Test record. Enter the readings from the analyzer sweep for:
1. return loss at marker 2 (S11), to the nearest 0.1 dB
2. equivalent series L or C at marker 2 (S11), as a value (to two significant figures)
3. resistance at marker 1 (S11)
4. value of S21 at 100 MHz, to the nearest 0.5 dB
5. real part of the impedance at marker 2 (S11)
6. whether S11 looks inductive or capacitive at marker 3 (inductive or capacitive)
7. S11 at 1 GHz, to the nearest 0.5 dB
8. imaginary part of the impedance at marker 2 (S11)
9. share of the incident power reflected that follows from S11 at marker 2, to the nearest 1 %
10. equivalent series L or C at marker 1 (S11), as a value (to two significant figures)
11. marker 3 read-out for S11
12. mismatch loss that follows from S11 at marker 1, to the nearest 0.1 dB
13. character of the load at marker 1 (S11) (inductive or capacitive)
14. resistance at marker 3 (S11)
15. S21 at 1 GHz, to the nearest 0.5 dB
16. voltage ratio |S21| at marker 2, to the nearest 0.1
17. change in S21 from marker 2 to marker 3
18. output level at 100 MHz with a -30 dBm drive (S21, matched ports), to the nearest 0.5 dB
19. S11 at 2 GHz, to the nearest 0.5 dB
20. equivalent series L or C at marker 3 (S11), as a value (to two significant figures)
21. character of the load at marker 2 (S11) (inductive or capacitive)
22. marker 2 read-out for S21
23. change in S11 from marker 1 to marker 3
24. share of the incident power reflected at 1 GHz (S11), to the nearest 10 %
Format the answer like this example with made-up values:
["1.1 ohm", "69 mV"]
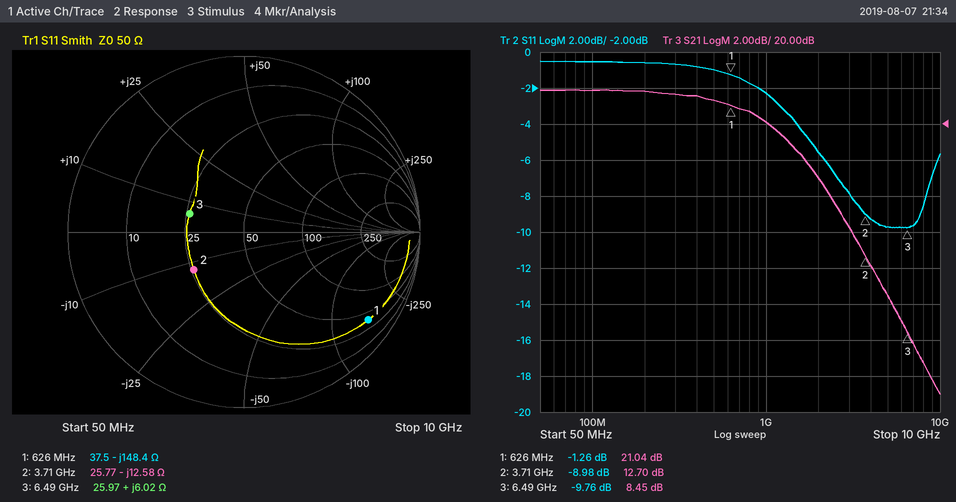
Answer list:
["9.0 dB", "3.4 pF", "37.5 Ω", "22.0 dB", "25.77 Ω", "inductive", "-2.5 dB", "-12.58 Ω", "13 %", "1.7 pF", "-9.76 dB", "6.0 dB", "capacitive", "25.97 Ω", "20.0 dB", "4.3", "-4.25 dB", "-8.0 dBm", "-5.5 dB", "150 pH", "capacitive", "12.70 dB", "-8.50 dB", "60 %"]
